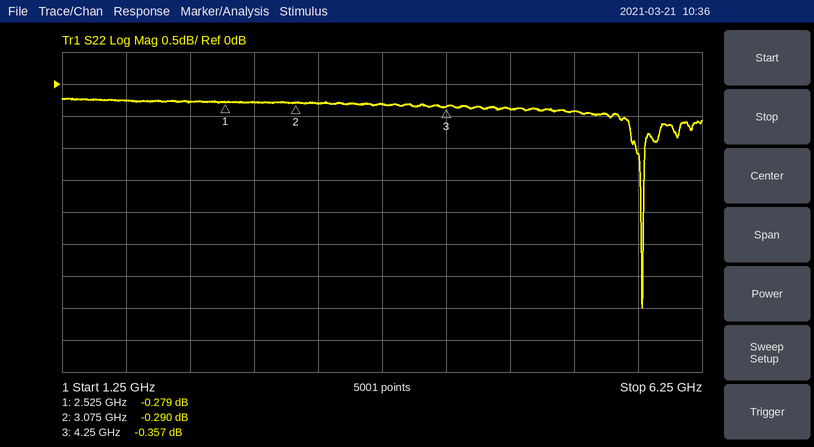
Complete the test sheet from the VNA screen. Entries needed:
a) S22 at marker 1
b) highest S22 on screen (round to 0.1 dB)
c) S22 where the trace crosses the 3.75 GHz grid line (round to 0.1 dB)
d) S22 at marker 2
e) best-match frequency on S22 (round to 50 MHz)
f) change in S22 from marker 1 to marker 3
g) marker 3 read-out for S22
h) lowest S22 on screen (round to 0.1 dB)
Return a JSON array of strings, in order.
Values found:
["-0.279 dB", "-0.2 dB", "-0.3 dB", "-0.290 dB", "5.80 GHz", "-0.078 dB", "-0.357 dB", "-3.5 dB"]
